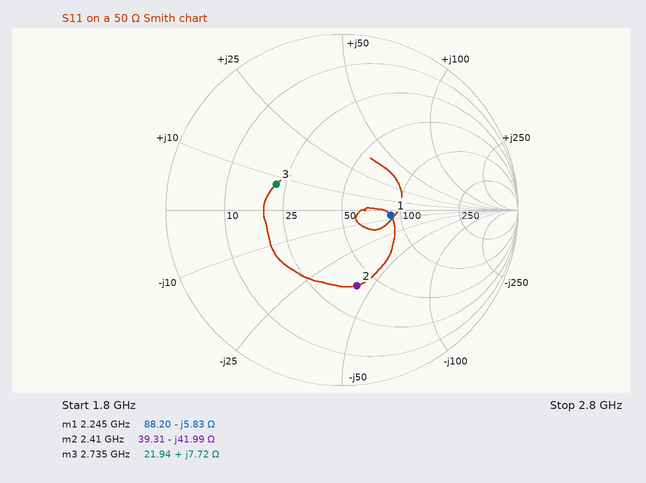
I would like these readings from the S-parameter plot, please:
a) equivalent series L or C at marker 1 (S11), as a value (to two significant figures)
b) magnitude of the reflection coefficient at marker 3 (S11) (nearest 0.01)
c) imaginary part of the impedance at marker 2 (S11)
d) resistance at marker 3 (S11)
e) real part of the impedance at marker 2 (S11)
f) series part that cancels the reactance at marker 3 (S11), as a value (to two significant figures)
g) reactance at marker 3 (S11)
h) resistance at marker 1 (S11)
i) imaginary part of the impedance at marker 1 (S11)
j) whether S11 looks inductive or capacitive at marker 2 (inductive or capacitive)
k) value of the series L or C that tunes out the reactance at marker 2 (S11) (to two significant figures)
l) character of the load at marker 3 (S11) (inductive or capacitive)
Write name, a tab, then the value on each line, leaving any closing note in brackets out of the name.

equivalent series L or C at marker 1 (S11), as a value	12 pF
magnitude of the reflection coefficient at marker 3 (S11)	0.40
imaginary part of the impedance at marker 2	-41.99 Ω
resistance at marker 3	21.94 Ω
real part of the impedance at marker 2	39.31 Ω
series part that cancels the reactance at marker 3 (S11), as a value	7.5 pF
reactance at marker 3	+7.72 Ω
resistance at marker 1	88.20 Ω
imaginary part of the impedance at marker 1	-5.83 Ω
whether S11 looks inductive or capacitive at marker 2	capacitive
value of the series L or C that tunes out the reactance at marker 2 (S11)	2.8 nH
character of the load at marker 3 (S11)	inductive
